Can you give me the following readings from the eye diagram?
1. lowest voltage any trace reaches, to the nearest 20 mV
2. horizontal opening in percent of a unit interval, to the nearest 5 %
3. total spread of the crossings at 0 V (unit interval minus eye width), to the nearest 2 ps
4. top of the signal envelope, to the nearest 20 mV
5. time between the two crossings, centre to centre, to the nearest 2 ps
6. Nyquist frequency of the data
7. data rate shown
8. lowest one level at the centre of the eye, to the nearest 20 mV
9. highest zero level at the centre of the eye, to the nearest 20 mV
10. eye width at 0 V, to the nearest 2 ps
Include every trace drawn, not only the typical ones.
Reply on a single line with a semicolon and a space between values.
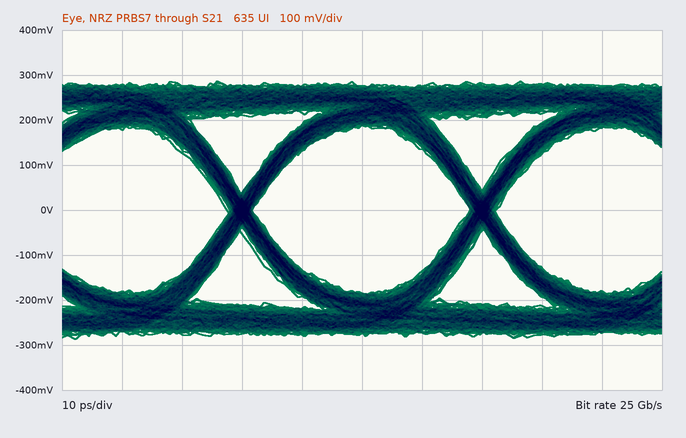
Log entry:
-280 mV; 90 %; 4 ps; 280 mV; 40 ps; 12.5 GHz; 25 Gb/s; 180 mV; -180 mV; 36 ps
